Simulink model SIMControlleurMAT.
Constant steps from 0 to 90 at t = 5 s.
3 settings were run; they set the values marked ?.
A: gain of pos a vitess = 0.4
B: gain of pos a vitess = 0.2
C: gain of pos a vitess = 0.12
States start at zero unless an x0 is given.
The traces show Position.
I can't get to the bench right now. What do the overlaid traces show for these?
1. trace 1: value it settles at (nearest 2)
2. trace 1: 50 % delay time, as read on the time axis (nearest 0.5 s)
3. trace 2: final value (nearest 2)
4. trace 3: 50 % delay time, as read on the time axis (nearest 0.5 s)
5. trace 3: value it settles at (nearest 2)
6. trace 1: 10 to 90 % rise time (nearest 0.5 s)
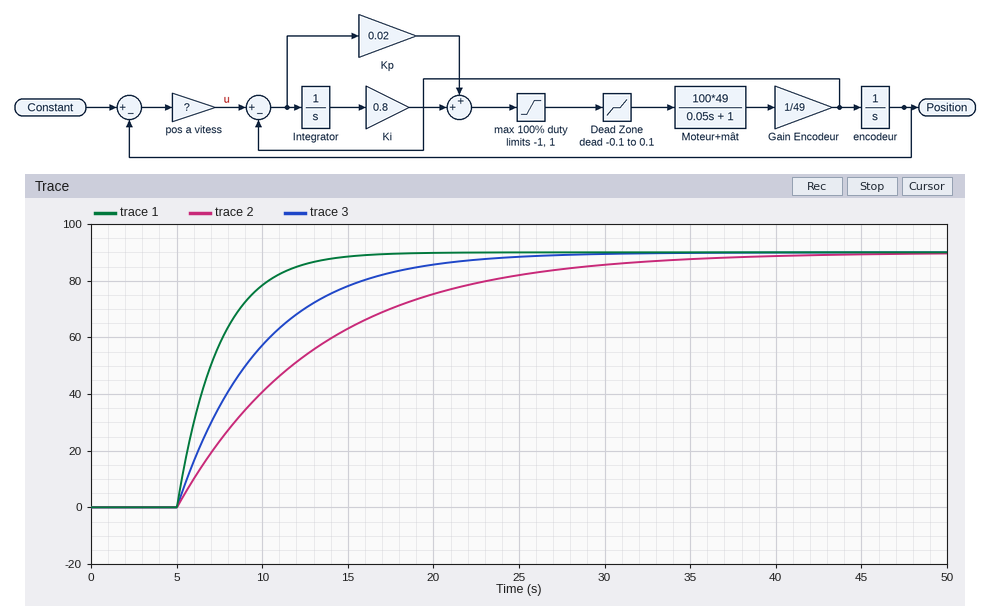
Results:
90
6.5 s
90
8.5 s
90
5.5 s
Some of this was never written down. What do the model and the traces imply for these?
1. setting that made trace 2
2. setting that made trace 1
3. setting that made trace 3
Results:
C
A
B
